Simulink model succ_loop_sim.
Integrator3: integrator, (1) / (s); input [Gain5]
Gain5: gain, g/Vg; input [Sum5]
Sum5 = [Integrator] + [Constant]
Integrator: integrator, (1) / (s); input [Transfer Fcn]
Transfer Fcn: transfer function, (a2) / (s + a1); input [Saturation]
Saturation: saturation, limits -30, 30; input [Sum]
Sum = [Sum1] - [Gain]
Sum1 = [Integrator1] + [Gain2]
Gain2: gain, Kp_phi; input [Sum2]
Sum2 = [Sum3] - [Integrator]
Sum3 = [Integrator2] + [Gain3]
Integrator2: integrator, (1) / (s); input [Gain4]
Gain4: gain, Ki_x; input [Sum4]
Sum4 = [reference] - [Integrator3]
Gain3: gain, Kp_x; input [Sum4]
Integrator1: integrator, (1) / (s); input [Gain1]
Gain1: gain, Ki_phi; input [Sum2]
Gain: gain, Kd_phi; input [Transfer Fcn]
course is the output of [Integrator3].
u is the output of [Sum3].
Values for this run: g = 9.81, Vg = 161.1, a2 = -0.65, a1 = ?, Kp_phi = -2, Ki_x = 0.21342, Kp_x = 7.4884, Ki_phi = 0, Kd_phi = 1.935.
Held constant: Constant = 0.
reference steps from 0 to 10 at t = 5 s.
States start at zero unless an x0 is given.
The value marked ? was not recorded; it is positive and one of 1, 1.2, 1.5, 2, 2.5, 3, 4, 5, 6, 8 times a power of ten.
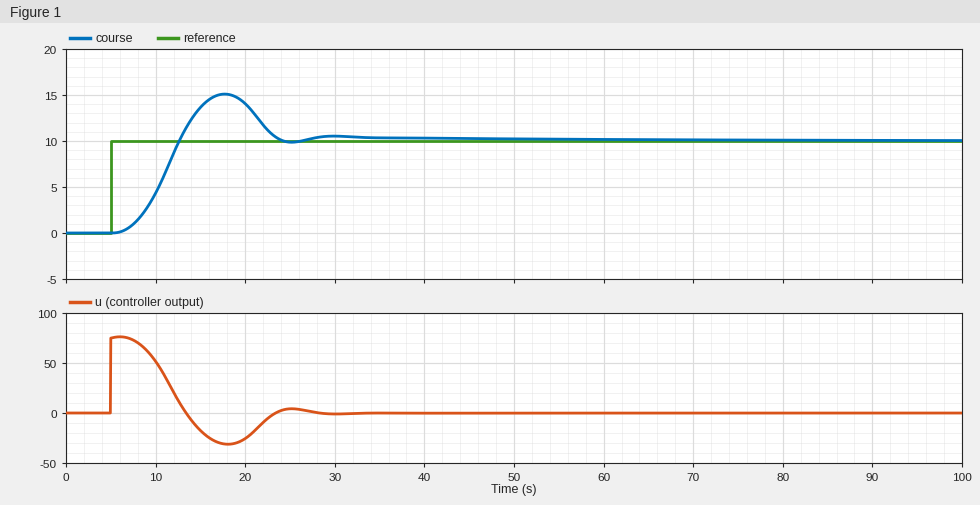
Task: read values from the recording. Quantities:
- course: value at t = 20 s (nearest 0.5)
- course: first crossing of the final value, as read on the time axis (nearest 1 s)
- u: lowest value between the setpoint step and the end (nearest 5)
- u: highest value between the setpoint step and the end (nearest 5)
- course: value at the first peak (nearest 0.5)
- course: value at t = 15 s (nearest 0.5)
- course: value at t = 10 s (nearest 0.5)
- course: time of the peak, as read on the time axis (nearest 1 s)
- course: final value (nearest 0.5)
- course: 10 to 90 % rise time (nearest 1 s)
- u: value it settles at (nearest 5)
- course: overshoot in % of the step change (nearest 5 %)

14.0
13 s
-30
75
15.0
13.5
4.5
18 s
10.0
5 s
0
50 %
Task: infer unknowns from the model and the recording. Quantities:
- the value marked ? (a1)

3
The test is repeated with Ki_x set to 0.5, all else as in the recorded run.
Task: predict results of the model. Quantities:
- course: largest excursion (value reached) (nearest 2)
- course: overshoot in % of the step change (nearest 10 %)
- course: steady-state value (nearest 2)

18
80 %
10
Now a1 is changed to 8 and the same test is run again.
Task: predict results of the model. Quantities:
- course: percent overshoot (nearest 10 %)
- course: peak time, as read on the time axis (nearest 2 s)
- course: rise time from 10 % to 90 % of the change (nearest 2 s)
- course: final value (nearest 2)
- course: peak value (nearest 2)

80 %
28 s
8 s
10
18
